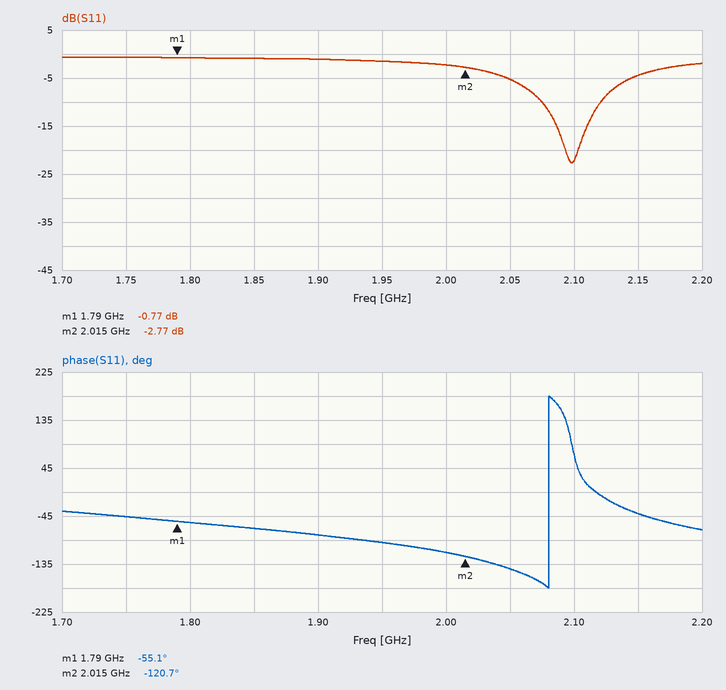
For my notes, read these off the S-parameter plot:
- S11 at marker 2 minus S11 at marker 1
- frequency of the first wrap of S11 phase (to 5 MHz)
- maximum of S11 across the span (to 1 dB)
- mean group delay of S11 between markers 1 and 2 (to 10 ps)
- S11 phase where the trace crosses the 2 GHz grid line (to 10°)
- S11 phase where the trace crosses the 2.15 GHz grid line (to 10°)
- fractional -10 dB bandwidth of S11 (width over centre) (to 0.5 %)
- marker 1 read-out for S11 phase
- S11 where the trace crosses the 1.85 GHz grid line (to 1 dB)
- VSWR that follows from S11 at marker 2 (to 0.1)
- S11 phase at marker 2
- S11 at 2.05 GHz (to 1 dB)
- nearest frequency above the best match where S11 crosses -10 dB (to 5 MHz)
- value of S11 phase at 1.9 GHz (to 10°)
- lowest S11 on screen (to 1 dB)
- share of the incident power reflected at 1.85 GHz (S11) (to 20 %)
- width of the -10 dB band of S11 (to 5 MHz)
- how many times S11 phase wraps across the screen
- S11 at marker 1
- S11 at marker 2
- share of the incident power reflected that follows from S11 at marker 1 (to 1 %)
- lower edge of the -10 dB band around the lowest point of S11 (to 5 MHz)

-2.00 dB
2.080 GHz
-1 dB
810 ps
-110°
-40°
2.0 %
-55.1°
-1 dB
6.3
-120.7°
-5 dB
2.120 GHz
-80°
-23 dB
80 %
45 MHz
1
-0.77 dB
-2.77 dB
84 %
2.075 GHz
